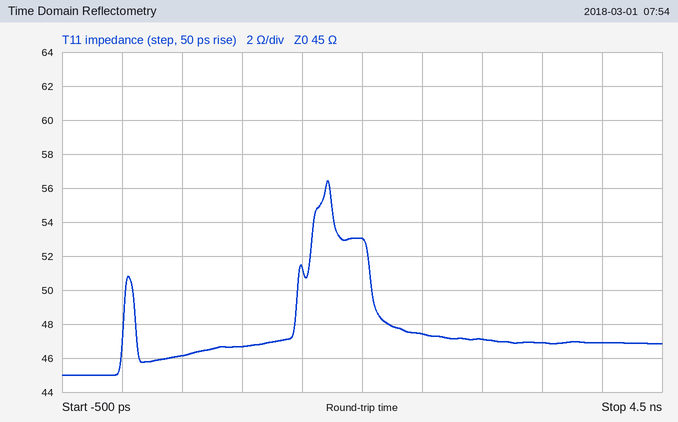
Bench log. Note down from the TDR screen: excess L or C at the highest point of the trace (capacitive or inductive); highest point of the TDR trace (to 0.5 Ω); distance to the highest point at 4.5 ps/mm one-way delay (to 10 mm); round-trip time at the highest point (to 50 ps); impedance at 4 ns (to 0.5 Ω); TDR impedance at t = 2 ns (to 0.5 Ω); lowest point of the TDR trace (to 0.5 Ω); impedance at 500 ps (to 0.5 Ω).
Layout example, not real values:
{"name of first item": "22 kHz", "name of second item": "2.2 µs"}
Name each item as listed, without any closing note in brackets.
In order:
{"excess L or C at the highest point of the trace": "inductive", "highest point of the TDR trace": "56.5 Ω", "distance to the highest point at 4.5 ps/mm one-way delay": "190 mm", "round-trip time at the highest point": "1.70 ns", "impedance at 4 ns": "47.0 Ω", "TDR impedance at t = 2 ns": "53.0 Ω", "lowest point of the TDR trace": "45.0 Ω", "impedance at 500 ps": "46.0 Ω"}
